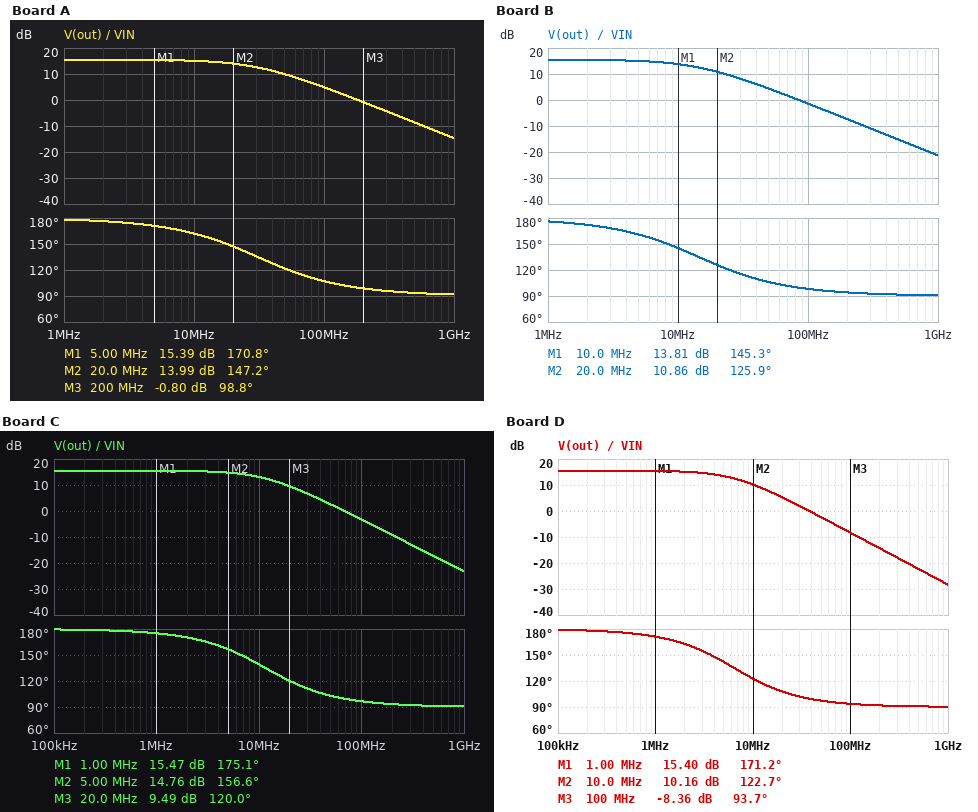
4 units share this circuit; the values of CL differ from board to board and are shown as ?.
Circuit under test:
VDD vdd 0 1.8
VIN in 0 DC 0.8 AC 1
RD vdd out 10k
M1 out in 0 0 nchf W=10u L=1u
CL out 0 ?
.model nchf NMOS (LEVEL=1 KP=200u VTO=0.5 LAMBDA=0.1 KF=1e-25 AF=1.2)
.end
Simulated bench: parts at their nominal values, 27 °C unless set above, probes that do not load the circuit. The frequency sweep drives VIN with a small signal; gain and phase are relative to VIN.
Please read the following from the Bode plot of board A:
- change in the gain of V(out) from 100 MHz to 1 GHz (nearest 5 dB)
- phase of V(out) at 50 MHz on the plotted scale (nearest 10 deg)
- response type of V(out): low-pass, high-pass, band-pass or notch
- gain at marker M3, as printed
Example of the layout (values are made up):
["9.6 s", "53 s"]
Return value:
["-20 dB", "120 deg", "low-pass", "-0.80 dB"]
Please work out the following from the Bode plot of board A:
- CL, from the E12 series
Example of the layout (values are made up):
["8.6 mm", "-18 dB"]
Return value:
["560 fF"]
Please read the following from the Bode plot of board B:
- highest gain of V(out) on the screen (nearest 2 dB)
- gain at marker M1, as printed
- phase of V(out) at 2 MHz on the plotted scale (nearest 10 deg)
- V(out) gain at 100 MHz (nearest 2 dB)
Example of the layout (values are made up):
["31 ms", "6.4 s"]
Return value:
["16 dB", "13.81 dB", "170 deg", "-2 dB"]
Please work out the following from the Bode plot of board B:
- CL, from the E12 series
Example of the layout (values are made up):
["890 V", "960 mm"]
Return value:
["1.2 pF"]
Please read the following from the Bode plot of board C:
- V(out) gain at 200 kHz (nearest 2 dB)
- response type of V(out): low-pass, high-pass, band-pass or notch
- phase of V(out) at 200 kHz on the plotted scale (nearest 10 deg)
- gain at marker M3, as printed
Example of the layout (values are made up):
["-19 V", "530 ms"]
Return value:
["16 dB", "low-pass", "180 deg", "9.49 dB"]
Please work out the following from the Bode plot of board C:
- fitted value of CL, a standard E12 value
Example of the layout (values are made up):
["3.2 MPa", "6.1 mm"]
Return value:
["1.5 pF"]
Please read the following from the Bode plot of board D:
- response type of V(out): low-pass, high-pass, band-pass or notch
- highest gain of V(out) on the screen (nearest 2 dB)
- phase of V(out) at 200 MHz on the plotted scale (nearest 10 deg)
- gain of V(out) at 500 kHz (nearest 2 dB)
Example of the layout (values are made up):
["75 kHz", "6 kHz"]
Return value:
["low-pass", "16 dB", "90 deg", "16 dB"]
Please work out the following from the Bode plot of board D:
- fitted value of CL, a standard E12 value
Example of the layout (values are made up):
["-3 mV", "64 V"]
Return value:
["2.7 pF"]
